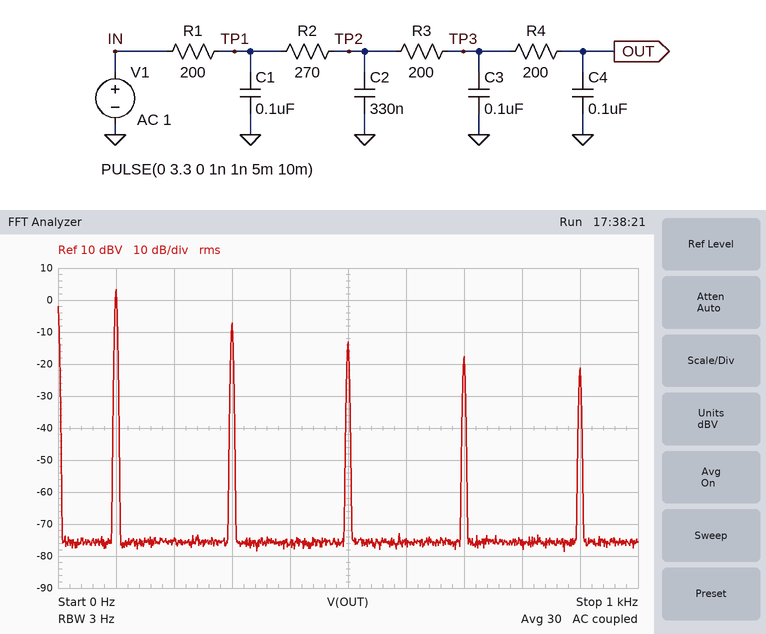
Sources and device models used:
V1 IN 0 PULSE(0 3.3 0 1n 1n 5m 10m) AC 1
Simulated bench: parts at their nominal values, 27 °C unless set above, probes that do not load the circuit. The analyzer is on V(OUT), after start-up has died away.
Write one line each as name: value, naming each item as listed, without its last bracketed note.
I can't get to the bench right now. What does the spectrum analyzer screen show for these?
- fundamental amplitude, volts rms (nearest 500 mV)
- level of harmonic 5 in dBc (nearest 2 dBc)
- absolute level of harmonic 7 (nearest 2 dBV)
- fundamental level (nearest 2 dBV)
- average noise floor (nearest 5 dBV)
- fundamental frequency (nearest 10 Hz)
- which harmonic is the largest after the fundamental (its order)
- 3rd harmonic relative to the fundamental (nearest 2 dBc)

fundamental amplitude, volts rms: 1.5 V
level of harmonic 5 in dBc: -16 dBc
absolute level of harmonic 7: -18 dBV
fundamental level: 4 dBV
average noise floor: -75 dBV
fundamental frequency: 100 Hz
which harmonic is the largest after the fundamental: 3
3rd harmonic relative to the fundamental: -10 dBc
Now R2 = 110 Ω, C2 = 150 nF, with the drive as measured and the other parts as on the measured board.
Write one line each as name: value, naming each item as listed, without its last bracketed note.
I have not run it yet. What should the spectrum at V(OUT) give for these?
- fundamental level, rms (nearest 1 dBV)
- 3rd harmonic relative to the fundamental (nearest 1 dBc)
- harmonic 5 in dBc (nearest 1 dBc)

fundamental level, rms: 3 dBV
3rd harmonic relative to the fundamental: -10 dBc
harmonic 5 in dBc: -15 dBc
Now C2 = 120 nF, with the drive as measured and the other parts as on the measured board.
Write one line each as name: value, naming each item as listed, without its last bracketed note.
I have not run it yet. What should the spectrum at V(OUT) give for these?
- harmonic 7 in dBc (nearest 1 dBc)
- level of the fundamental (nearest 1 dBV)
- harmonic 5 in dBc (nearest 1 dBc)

harmonic 7 in dBc: -19 dBc
level of the fundamental: 3 dBV
harmonic 5 in dBc: -15 dBc
